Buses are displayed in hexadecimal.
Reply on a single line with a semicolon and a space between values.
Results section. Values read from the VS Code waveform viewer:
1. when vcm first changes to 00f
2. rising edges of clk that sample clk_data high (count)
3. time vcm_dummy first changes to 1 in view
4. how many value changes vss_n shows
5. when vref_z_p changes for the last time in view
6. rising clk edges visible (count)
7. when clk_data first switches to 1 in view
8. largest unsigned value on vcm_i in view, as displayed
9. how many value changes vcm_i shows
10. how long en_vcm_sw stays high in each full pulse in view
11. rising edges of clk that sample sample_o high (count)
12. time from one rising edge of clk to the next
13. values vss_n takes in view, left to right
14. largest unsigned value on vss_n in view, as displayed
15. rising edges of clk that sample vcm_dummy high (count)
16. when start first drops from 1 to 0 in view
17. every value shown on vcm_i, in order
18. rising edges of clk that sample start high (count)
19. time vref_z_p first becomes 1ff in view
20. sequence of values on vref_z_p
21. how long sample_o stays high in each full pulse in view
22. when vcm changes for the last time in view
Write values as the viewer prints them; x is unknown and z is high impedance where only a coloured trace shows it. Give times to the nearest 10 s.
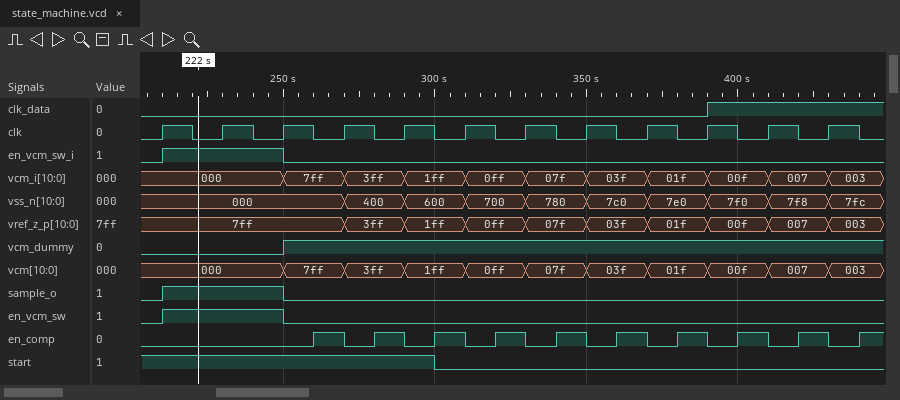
390 s; 2; 250 s; 9; 430 s; 12; 390 s; 7ff; 10; 40 s; 2; 20 s; 000, 400, 600, 700, 780, 7c0, 7e0, 7f0, 7f8, 7fc; 7fc; 9; 300 s; 000, 7ff, 3ff, 1ff, 0ff, 07f, 03f, 01f, 00f, 007, 003; 5; 290 s; 7ff, 3ff, 1ff, 0ff, 07f, 03f, 01f, 00f, 007, 003; 40 s; 430 s
